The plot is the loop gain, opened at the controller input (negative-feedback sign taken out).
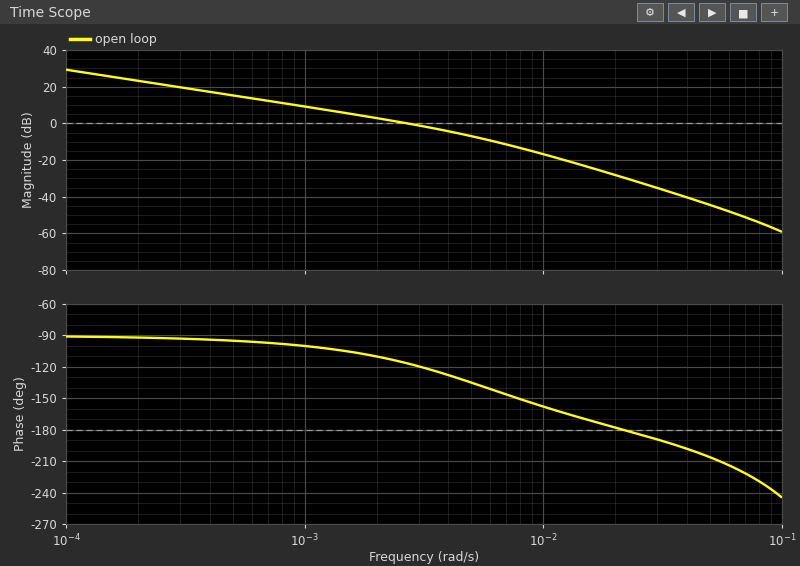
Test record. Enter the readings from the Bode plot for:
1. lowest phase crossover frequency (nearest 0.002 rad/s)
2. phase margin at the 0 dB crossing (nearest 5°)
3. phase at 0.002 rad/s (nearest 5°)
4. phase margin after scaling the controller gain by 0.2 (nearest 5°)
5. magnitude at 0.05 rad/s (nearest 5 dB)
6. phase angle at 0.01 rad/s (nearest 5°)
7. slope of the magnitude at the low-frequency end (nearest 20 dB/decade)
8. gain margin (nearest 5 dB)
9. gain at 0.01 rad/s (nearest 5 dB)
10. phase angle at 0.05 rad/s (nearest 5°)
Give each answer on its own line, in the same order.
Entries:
0.022 rad/s
65°
-110°
85°
-45 dB
-160°
-20 dB/decade
30 dB
-15 dB
-205°
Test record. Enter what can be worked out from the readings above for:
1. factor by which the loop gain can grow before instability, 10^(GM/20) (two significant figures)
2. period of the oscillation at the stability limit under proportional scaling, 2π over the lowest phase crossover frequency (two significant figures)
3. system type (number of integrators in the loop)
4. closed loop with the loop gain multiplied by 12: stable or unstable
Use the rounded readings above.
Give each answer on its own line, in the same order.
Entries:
32
290 s
1
stable
